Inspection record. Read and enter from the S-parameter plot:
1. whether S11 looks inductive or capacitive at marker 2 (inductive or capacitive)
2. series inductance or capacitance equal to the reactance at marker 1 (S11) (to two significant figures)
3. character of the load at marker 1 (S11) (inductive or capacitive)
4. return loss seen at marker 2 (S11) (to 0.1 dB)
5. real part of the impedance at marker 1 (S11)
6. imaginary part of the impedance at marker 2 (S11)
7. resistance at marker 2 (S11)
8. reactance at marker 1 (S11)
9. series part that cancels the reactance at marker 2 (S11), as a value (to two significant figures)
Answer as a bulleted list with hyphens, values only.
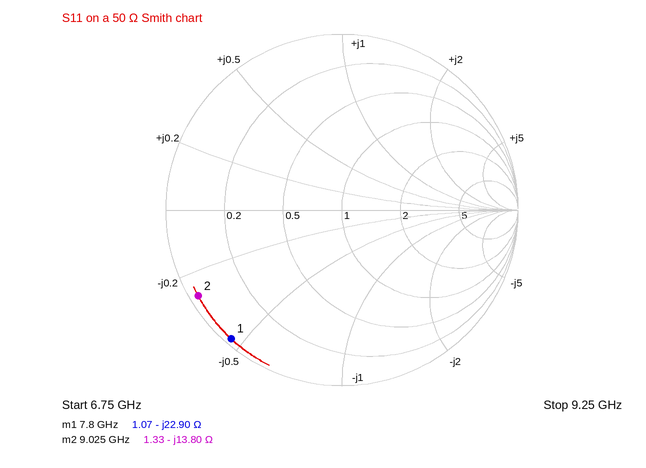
- capacitive
- 890 fF
- capacitive
- 0.4 dB
- 1.07 Ω
- -13.80 Ω
- 1.33 Ω
- -22.90 Ω
- 240 pH
